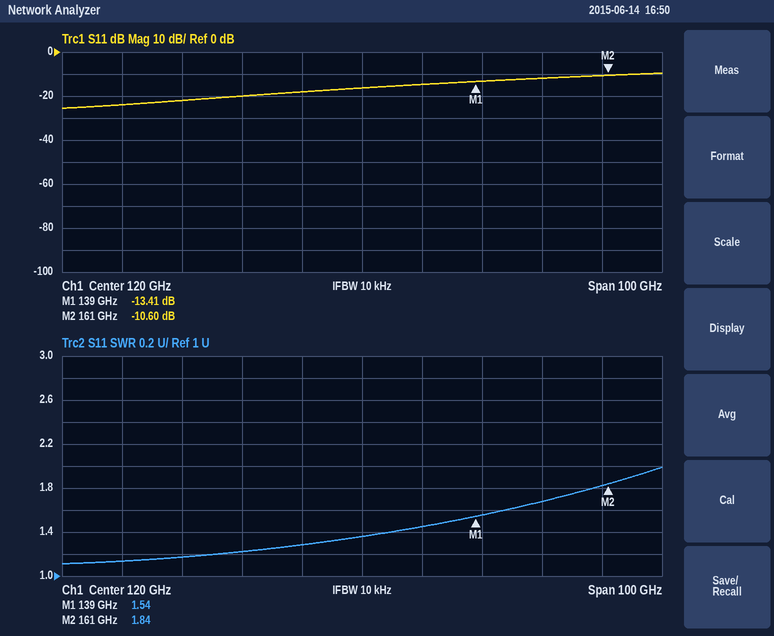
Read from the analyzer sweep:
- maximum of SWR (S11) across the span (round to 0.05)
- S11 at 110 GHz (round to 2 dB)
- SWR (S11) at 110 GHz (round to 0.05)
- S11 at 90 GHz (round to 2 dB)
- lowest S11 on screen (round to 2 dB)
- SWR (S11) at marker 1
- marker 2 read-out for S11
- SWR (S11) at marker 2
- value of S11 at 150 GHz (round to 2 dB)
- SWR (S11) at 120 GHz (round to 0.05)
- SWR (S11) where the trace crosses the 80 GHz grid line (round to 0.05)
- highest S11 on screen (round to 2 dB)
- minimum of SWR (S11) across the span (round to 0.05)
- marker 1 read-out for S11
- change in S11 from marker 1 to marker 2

2.00
-18 dB
1.30
-22 dB
-26 dB
1.54
-10.60 dB
1.84
-12 dB
1.35
1.15
-10 dB
1.10
-13.41 dB
2.81 dB
